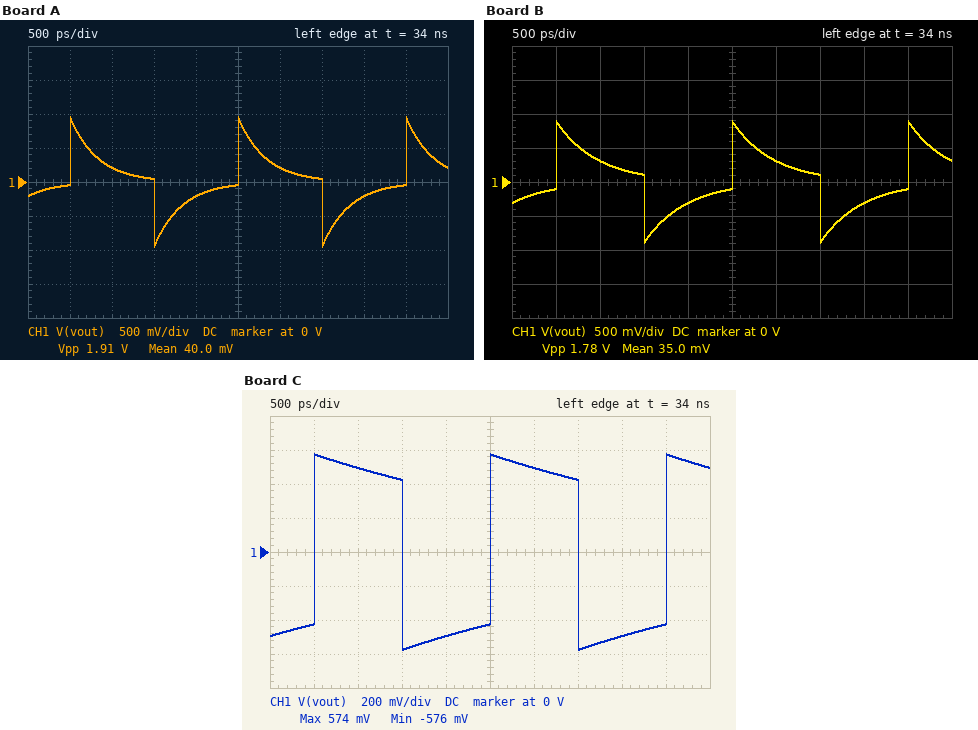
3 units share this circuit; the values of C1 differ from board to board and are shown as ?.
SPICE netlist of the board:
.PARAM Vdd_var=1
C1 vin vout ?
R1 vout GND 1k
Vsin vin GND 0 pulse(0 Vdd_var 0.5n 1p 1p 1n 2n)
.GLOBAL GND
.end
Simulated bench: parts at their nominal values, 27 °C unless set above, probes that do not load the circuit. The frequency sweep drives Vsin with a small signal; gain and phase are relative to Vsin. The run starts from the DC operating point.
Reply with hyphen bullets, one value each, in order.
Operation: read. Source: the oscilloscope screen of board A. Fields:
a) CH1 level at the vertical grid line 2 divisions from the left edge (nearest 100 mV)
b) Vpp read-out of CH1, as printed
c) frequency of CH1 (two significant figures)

- 200 mV
- 1.91 V
- 500 MHz
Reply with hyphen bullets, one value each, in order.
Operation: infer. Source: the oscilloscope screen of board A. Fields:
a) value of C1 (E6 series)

- 330 fF
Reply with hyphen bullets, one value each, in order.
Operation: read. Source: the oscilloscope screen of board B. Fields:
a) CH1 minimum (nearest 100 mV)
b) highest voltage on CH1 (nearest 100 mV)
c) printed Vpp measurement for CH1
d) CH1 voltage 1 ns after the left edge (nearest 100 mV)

- -900 mV
- 900 mV
- 1.78 V
- 300 mV
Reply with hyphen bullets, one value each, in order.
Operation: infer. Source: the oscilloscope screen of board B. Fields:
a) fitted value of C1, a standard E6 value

- 470 fF
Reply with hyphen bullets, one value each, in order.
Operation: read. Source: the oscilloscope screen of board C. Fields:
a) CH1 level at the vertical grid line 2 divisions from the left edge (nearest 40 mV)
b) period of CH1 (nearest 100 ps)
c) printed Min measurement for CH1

- 480 mV
- 2.0 ns
- -576 mV
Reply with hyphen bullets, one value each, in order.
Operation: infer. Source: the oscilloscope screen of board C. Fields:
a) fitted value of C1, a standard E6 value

- 3.3 pF
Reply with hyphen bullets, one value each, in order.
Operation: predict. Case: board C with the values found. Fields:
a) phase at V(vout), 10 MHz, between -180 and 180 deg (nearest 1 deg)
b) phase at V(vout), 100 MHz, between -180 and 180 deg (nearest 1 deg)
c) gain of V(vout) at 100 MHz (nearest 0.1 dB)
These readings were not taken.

- 78 deg
- 26 deg
- -0.9 dB
